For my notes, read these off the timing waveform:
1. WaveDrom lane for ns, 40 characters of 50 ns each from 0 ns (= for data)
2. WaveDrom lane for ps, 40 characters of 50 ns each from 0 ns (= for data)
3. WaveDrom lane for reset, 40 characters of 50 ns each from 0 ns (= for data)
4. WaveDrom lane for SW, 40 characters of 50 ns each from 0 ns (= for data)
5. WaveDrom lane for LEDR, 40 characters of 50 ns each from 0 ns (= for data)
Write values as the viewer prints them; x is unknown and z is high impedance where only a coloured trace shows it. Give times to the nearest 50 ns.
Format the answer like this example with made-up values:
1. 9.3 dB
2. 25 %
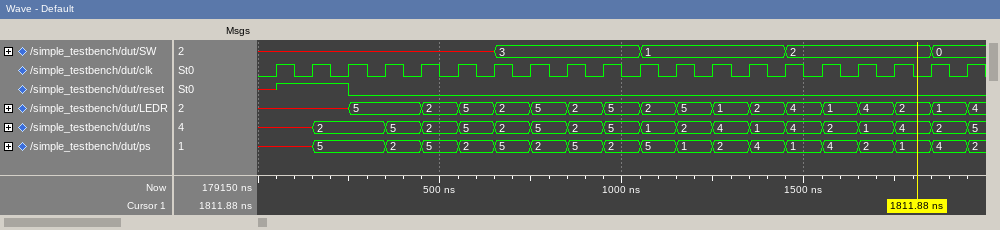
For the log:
1. {name: 'ns', wave: 'x..=...=.=.=.=.=.=.=.=.=.=.=.=.=.=.=.=.=', data: '2 5 2 5 2 5 2 5 1 2 4 1 4 2 1 4 2 5'}
2. {name: 'ps', wave: 'x..=...=.=.=.=.=.=.=.=.=.=.=.=.=.=.=.=.=', data: '5 2 5 2 5 2 5 2 5 1 2 4 1 4 2 1 4 2'}
3. {name: 'reset', wave: 'x1...0..................................'}
4. {name: 'SW', wave: 'x............=.......=.......=.......=..', data: '3 1 2 0'}
5. {name: 'LEDR', wave: 'x....=...=.=.=.=.=.=.=.=.=.=.=.=.=.=.=.=', data: '5 2 5 2 5 2 5 2 5 1 2 4 1 4 2 1 4'}
